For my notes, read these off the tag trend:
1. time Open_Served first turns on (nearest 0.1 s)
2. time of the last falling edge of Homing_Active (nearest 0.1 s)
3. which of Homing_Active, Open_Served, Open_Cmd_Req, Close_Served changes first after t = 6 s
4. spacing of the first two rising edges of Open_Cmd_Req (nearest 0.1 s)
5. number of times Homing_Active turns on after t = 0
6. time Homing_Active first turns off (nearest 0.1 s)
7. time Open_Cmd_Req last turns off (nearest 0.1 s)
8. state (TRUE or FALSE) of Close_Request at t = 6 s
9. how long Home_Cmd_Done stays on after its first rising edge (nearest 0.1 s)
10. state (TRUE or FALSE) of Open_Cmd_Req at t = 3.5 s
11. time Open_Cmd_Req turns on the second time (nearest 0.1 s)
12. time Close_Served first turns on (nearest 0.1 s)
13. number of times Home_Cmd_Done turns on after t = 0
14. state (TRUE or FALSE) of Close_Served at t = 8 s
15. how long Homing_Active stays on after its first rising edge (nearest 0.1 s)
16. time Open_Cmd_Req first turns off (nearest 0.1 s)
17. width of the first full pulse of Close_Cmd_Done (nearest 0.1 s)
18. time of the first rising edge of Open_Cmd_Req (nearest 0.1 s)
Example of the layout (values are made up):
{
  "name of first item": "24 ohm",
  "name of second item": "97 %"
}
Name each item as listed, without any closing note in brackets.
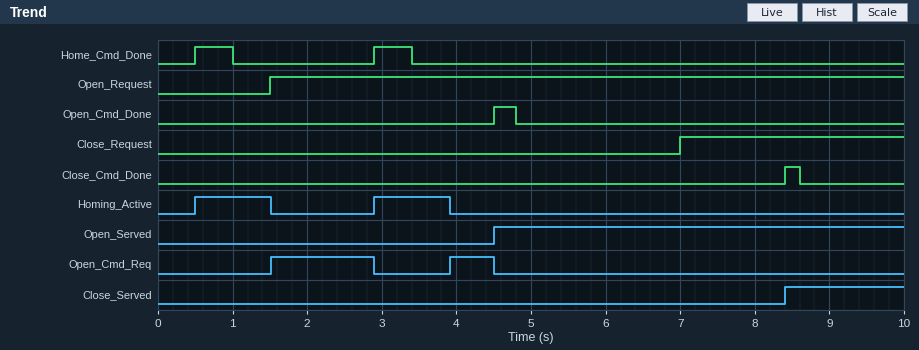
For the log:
{
  "time Open_Served first turns on": "4.5 s",
  "time of the last falling edge of Homing_Active": "3.9 s",
  "which of Homing_Active, Open_Served, Open_Cmd_Req, Close_Served changes first after t = 6 s": "Close_Served",
  "spacing of the first two rising edges of Open_Cmd_Req": "2.4 s",
  "number of times Homing_Active turns on after t = 0": "2",
  "time Homing_Active first turns off": "1.5 s",
  "time Open_Cmd_Req last turns off": "4.5 s",
  "state (TRUE or FALSE) of Close_Request at t = 6 s": "FALSE",
  "how long Home_Cmd_Done stays on after its first rising edge": "0.5 s",
  "state (TRUE or FALSE) of Open_Cmd_Req at t = 3.5 s": "FALSE",
  "time Open_Cmd_Req turns on the second time": "3.9 s",
  "time Close_Served first turns on": "8.4 s",
  "number of times Home_Cmd_Done turns on after t = 0": "2",
  "state (TRUE or FALSE) of Close_Served at t = 8 s": "FALSE",
  "how long Homing_Active stays on after its first rising edge": "1.0 s",
  "time Open_Cmd_Req first turns off": "2.9 s",
  "width of the first full pulse of Close_Cmd_Done": "0.2 s",
  "time of the first rising edge of Open_Cmd_Req": "1.5 s"
}
